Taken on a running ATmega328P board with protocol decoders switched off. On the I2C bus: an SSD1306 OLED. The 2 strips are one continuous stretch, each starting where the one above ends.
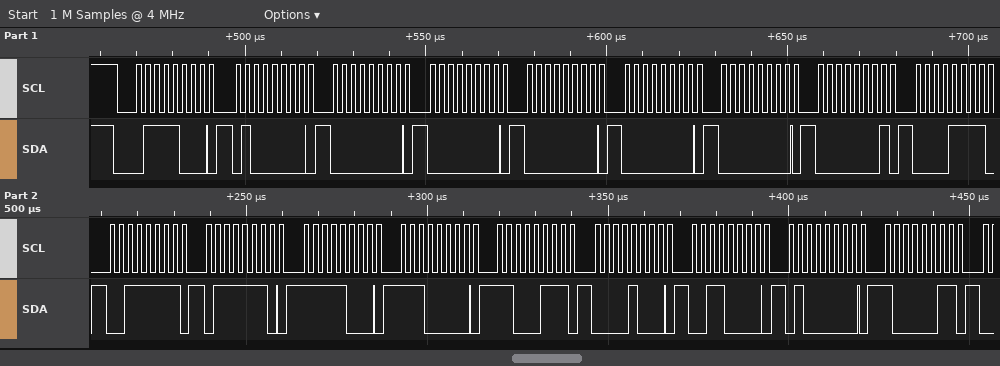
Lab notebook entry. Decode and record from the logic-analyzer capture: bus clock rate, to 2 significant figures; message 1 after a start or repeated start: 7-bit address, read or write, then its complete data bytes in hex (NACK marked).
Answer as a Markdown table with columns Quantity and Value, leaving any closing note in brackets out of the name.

| Quantity | Value |
|---|---|
| bus clock rate, to 2 significant figures | 400 kHz |
| message 1 after a start or repeated start: 7-bit address, read or write, then its complete data bytes in hex | 0x3C write: 40 00 00 00 00 00 01 0F 3F 7E F8 E0 C7 08 30 40 83 |
